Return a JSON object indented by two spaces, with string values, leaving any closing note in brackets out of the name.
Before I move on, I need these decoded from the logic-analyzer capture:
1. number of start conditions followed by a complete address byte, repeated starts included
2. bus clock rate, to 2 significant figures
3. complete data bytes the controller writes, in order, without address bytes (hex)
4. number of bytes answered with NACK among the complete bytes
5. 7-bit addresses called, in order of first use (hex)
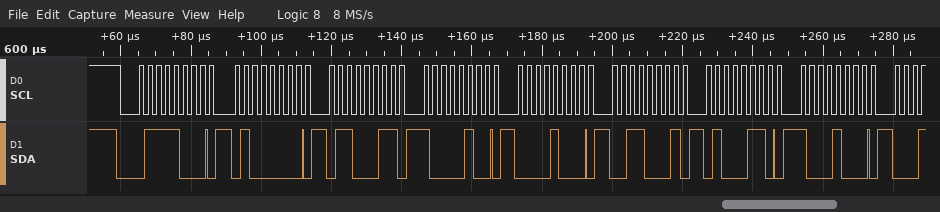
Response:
{
  "number of start conditions followed by a complete address byte, repeated starts included": "1",
  "bus clock rate, to 2 significant figures": "400 kHz",
  "complete data bytes the controller writes, in order, without address bytes": "40 63 84 08 31 46 88",
  "number of bytes answered with NACK among the complete bytes": "0",
  "7-bit addresses called, in order of first use": "0x3C"
}
